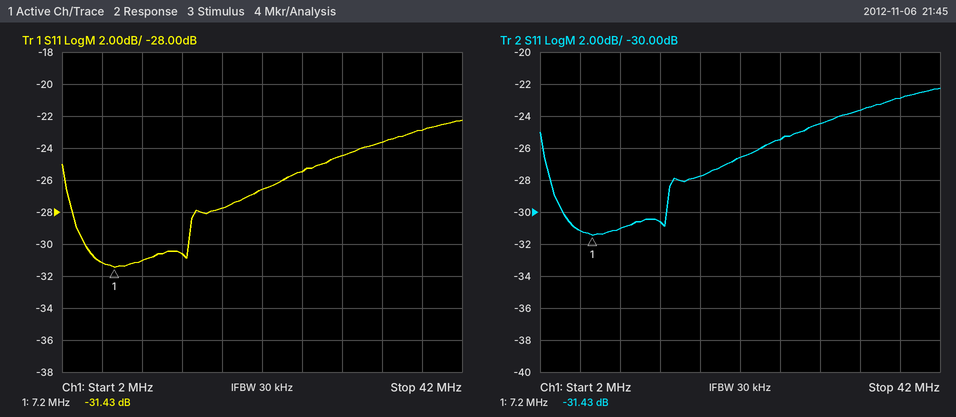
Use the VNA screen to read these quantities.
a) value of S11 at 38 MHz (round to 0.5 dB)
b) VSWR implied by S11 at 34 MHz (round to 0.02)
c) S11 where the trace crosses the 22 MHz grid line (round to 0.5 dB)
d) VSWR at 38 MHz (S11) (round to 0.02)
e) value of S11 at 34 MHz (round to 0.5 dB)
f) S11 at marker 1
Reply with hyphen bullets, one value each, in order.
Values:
- -23.0 dB
- 1.14
- -26.5 dB
- 1.16
- -23.5 dB
- -31.43 dB
